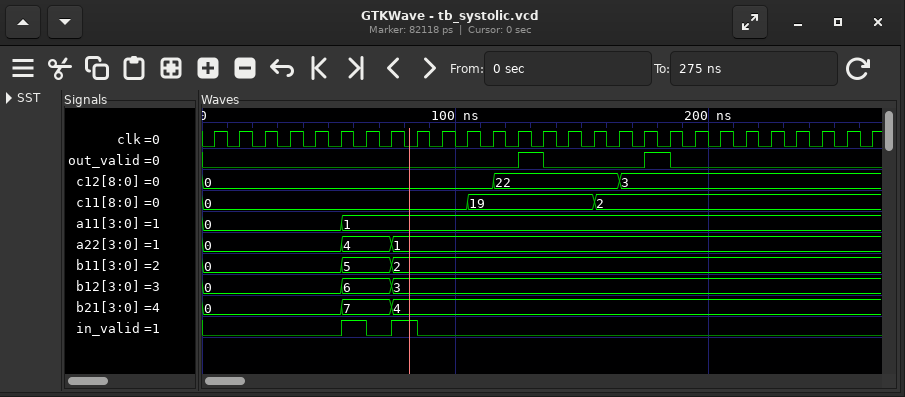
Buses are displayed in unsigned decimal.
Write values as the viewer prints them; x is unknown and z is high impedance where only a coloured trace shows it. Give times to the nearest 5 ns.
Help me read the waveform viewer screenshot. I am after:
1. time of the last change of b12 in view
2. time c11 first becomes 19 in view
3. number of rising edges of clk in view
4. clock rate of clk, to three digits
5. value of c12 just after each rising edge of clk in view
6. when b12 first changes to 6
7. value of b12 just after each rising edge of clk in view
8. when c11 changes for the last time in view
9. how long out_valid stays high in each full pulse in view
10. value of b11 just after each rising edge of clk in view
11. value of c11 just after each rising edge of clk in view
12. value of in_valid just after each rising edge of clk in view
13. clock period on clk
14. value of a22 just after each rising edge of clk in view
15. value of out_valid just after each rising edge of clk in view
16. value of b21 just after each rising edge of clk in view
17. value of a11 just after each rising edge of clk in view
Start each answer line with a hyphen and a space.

- 75 ns
- 105 ns
- 27
- 100 MHz
- 0, 0, 0, 0, 0, 0, 0, 0, 0, 0, 0, 22, 22, 22, 22, 22, 3, 3, 3, 3, 3, 3, 3, 3, 3, 3, 3
- 55 ns
- 0, 0, 0, 0, 0, 6, 6, 3, 3, 3, 3, 3, 3, 3, 3, 3, 3, 3, 3, 3, 3, 3, 3, 3, 3, 3, 3
- 155 ns
- 10 ns, 10 ns
- 0, 0, 0, 0, 0, 5, 5, 2, 2, 2, 2, 2, 2, 2, 2, 2, 2, 2, 2, 2, 2, 2, 2, 2, 2, 2, 2
- 0, 0, 0, 0, 0, 0, 0, 0, 0, 0, 19, 19, 19, 19, 19, 2, 2, 2, 2, 2, 2, 2, 2, 2, 2, 2, 2
- 0 0 0 0 0 1 0 1 0 0 0 0 0 0 0 0 0 0 0 0 0 0 0 0 0 0 0
- 10 ns
- 0, 0, 0, 0, 0, 4, 4, 1, 1, 1, 1, 1, 1, 1, 1, 1, 1, 1, 1, 1, 1, 1, 1, 1, 1, 1, 1
- 0 0 0 0 0 0 0 0 0 0 0 0 1 0 0 0 0 1 0 0 0 0 0 0 0 0 0
- 0, 0, 0, 0, 0, 7, 7, 4, 4, 4, 4, 4, 4, 4, 4, 4, 4, 4, 4, 4, 4, 4, 4, 4, 4, 4, 4
- 0, 0, 0, 0, 0, 1, 1, 1, 1, 1, 1, 1, 1, 1, 1, 1, 1, 1, 1, 1, 1, 1, 1, 1, 1, 1, 1
